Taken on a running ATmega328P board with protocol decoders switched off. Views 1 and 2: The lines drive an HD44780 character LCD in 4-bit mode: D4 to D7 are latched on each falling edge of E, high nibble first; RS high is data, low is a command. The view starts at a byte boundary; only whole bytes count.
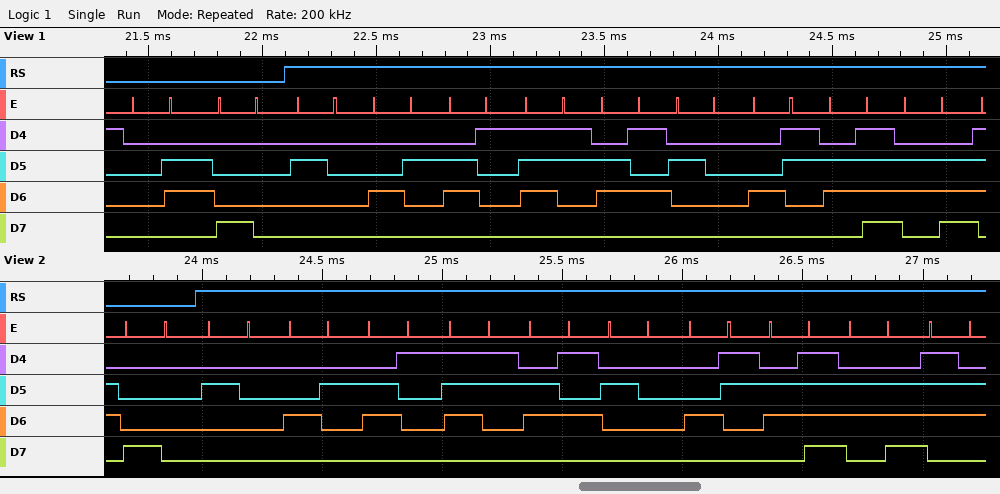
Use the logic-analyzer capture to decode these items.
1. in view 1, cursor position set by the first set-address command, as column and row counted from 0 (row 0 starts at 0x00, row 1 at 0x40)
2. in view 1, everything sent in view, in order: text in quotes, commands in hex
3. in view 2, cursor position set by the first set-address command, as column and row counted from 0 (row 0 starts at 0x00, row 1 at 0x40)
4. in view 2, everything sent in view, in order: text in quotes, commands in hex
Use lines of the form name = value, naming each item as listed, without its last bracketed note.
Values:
in view 1, cursor position set by the first set-address command, as column and row counted from 0 = column 0, row 0
in view 1, everything sent in view, in order: text in quotes, commands in hex = 0x06 0x80 " Base Con"
in view 2, cursor position set by the first set-address command, as column and row counted from 0 = column 0, row 0
in view 2, everything sent in view, in order: text in quotes, commands in hex = 0x80 " Base Conv"
